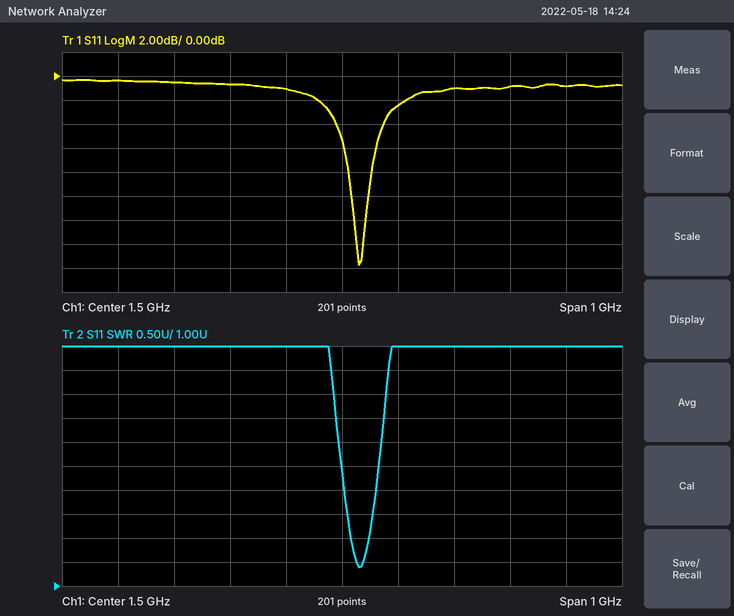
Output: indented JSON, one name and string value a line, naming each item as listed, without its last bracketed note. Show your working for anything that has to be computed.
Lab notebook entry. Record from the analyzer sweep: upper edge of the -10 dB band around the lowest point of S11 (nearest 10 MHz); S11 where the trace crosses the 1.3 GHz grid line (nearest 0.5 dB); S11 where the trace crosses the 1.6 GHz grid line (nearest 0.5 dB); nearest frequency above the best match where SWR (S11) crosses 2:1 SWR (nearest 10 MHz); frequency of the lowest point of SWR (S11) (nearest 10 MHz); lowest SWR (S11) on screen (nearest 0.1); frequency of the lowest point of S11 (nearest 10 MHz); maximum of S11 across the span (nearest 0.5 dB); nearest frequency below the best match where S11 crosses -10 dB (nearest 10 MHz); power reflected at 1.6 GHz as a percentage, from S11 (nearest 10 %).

{
  "upper edge of the -10 dB band around the lowest point of S11": "1.55 GHz",
  "S11 where the trace crosses the 1.3 GHz grid line": "-0.5 dB",
  "S11 where the trace crosses the 1.6 GHz grid line": "-2.5 dB",
  "nearest frequency above the best match where SWR (S11) crosses 2:1 SWR": "1.55 GHz",
  "frequency of the lowest point of SWR (S11)": "1.53 GHz",
  "lowest SWR (S11) on screen": "1.4",
  "frequency of the lowest point of S11": "1.53 GHz",
  "maximum of S11 across the span": "-0.5 dB",
  "nearest frequency below the best match where S11 crosses -10 dB": "1.52 GHz",
  "power reflected at 1.6 GHz as a percentage, from S11": "10^(-2.5/10) ≈ 56.2 %, so 60 % to the nearest 10 %"
}
